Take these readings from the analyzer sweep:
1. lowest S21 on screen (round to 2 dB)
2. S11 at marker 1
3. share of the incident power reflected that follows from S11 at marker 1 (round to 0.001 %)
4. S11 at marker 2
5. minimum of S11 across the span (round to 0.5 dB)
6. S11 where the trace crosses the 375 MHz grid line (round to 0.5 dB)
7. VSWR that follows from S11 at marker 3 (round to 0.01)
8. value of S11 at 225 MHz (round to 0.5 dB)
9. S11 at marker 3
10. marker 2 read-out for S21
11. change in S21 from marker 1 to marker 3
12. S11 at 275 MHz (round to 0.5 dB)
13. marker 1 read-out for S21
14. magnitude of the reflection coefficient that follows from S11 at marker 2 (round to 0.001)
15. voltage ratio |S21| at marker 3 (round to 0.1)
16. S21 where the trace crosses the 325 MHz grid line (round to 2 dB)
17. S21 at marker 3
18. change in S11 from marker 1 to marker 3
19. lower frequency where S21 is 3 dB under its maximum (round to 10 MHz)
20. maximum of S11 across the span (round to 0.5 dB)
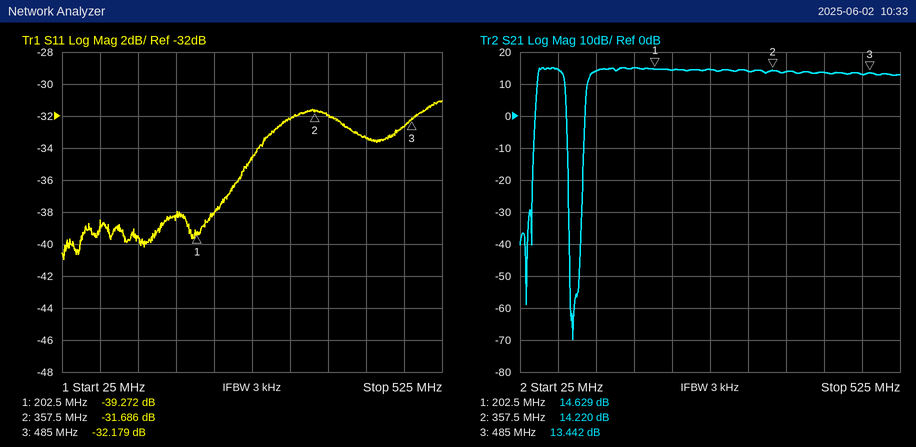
-70 dB
-39.272 dB
0.012 %
-31.686 dB
-41.0 dB
-32.0 dB
1.05
-38.0 dB
-32.179 dB
14.220 dB
-1.187 dB
-34.5 dB
14.629 dB
0.026
4.7
14 dB
13.442 dB
7.093 dB
50 MHz
-31.0 dB
